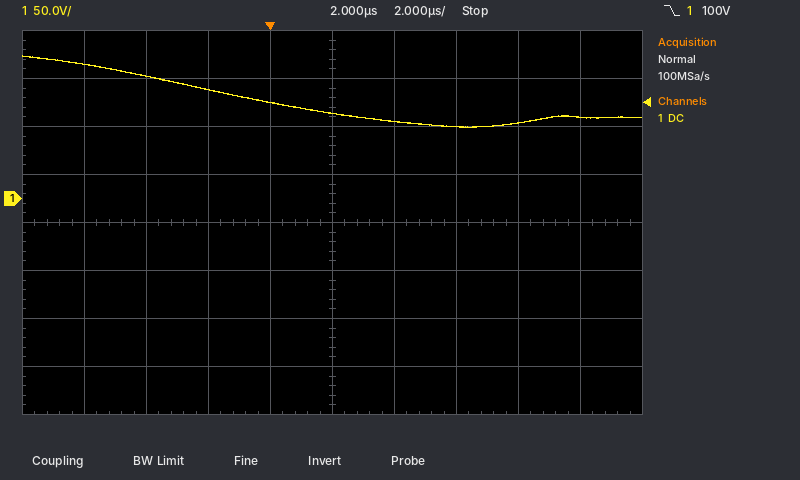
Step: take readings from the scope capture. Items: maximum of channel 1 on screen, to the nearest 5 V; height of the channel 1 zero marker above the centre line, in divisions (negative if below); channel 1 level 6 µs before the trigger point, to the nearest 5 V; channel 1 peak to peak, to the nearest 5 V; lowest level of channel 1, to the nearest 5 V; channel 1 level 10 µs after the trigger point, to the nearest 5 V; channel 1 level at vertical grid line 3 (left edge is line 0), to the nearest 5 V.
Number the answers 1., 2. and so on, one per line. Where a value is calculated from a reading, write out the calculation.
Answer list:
1. 150 V
2. +0.5 div
3. 140 V
4. 150 V − (75 V) = 75 V
5. 75 V
6. 85 V
7. 115 V
